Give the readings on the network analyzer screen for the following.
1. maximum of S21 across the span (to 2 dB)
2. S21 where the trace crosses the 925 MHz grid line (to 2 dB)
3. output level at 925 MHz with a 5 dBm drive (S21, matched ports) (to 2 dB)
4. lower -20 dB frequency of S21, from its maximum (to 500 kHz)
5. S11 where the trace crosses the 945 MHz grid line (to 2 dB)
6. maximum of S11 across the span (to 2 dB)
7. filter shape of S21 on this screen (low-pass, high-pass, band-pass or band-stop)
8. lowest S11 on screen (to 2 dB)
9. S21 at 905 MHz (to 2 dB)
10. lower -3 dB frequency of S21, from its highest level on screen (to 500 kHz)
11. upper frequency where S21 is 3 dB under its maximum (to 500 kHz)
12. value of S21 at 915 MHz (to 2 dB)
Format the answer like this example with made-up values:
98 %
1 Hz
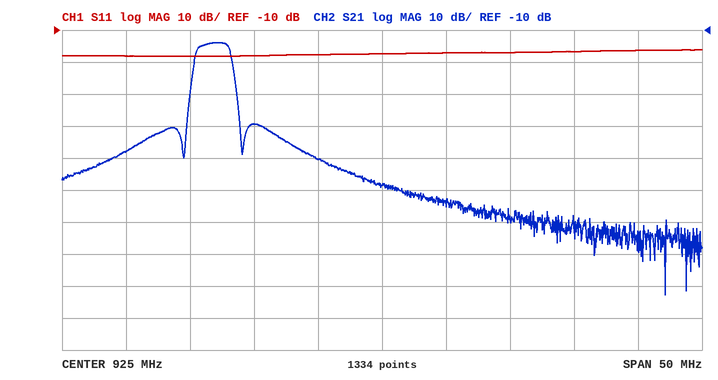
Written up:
-14 dB
-58 dB
-54 dBm
910.0 MHz
-16 dB
-16 dB
band-pass
-18 dB
-48 dB
910.5 MHz
913.0 MHz
-40 dB
